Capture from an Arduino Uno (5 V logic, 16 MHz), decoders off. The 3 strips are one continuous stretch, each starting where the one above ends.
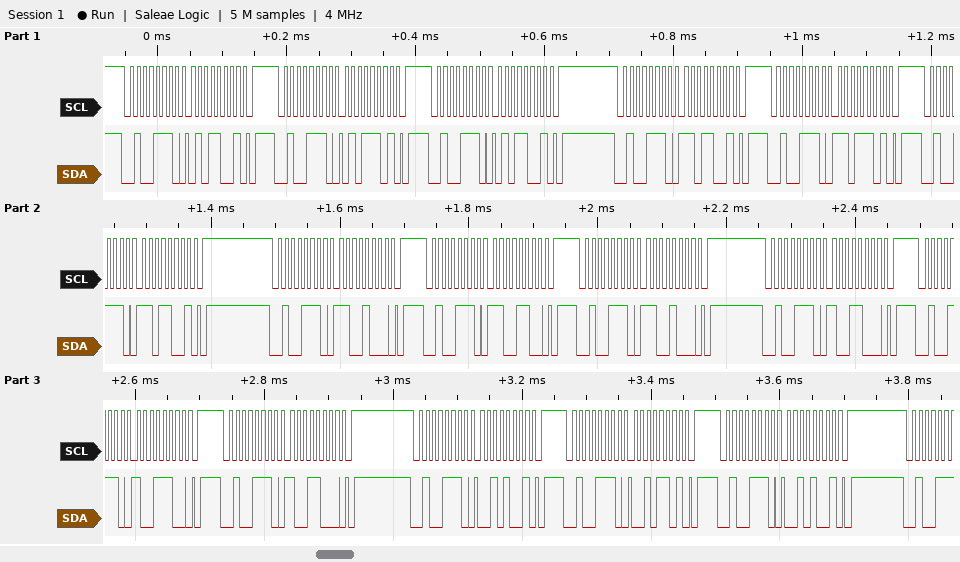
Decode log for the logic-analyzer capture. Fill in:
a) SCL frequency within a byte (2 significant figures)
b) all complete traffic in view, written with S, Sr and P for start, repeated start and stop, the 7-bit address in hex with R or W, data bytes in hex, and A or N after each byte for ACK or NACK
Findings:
100 kHz
S 27W A 59 A P S 27W A 5D A P S 27W A 59 A P S 27W A D9 A P S 27W A DD A P S 27W A D9 A P S 27W A C8 A P S 27W A CC A P S 27W A C8 A P S 27W A 98 A P S 27W A 9C A P S 27W A 98 A P S 27W A 29 A P S 27W A 2D A P S 27W A 29 A P
